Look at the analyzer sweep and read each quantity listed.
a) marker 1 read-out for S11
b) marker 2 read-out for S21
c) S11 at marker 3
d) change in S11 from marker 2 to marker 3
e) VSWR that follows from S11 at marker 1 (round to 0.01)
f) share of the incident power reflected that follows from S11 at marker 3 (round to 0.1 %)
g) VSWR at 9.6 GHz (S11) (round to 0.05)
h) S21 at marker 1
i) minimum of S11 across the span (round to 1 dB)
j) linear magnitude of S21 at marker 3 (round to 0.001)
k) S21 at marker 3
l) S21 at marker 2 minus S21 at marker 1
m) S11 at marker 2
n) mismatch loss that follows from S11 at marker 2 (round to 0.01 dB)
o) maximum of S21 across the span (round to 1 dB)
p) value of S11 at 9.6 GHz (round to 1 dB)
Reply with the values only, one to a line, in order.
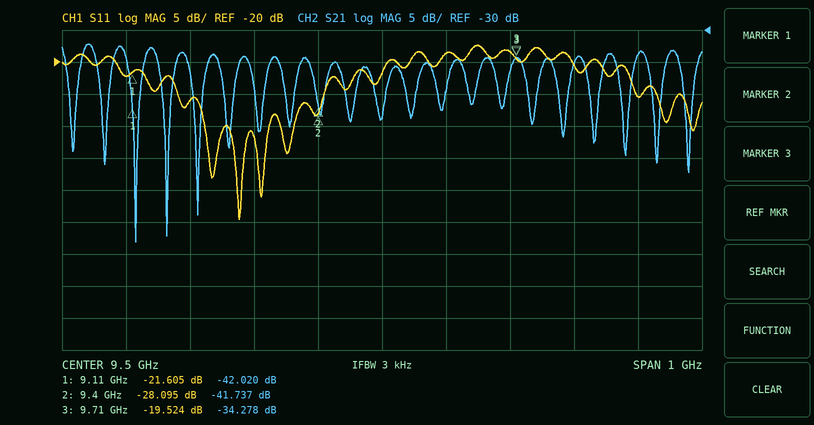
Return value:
-21.605 dB
-41.737 dB
-19.524 dB
8.571 dB
1.18
1.1 %
1.25
-42.020 dB
-45 dB
0.019
-34.278 dB
0.283 dB
-28.095 dB
0.01 dB
-32 dB
-19 dB
